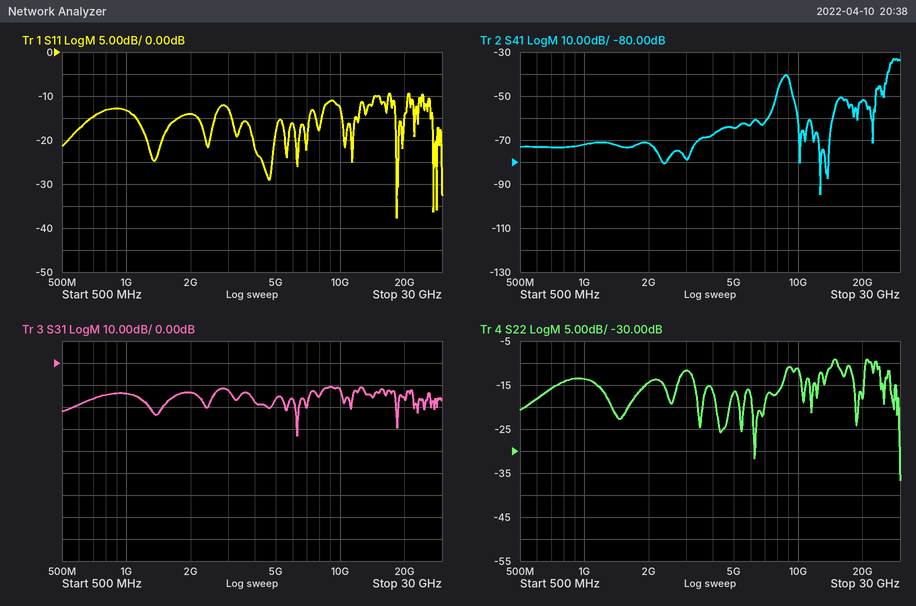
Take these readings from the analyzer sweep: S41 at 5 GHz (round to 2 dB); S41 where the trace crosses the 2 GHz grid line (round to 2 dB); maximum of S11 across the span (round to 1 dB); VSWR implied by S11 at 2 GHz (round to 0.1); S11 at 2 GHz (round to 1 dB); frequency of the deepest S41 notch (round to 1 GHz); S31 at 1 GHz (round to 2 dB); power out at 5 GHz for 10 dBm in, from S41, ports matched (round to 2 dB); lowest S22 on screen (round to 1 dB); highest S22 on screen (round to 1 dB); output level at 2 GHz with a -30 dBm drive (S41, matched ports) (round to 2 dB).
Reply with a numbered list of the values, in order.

1. -64 dB
2. -72 dB
3. -9 dB
4. 1.5
5. -14 dB
6. 13 GHz
7. -14 dB
8. -54 dBm
9. -37 dB
10. -9 dB
11. -102 dBm
